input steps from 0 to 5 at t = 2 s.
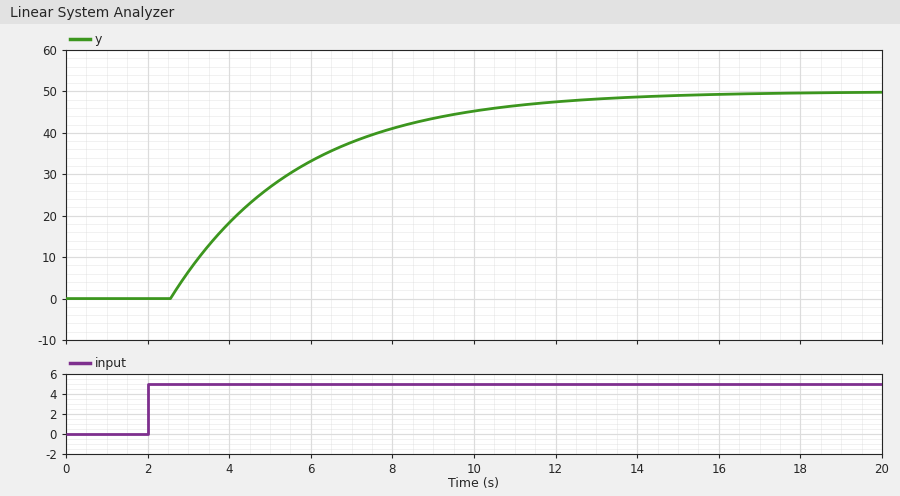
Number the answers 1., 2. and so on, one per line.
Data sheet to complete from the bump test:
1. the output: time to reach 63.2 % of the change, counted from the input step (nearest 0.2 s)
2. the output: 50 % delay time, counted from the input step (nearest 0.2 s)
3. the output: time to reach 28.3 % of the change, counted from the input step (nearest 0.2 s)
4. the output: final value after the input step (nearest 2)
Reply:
1. 3.8 s
2. 2.8 s
3. 1.6 s
4. 50
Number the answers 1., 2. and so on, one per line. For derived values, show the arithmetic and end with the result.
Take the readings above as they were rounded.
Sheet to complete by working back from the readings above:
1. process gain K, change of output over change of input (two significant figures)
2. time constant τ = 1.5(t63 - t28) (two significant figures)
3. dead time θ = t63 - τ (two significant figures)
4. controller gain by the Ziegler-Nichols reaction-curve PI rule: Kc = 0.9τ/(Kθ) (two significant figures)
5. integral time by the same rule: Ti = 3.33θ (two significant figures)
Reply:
1. (50 - 0) / 5 = 10
2. 1.5 × (3.8 - 1.6) = 3.3 s
3. 3.8 - 3.3 = 0.50 s
4. 0.9 × 3.3 / (10 × 0.5) = 0.59
5. 3.33 × 0.5 = 1.7 s
